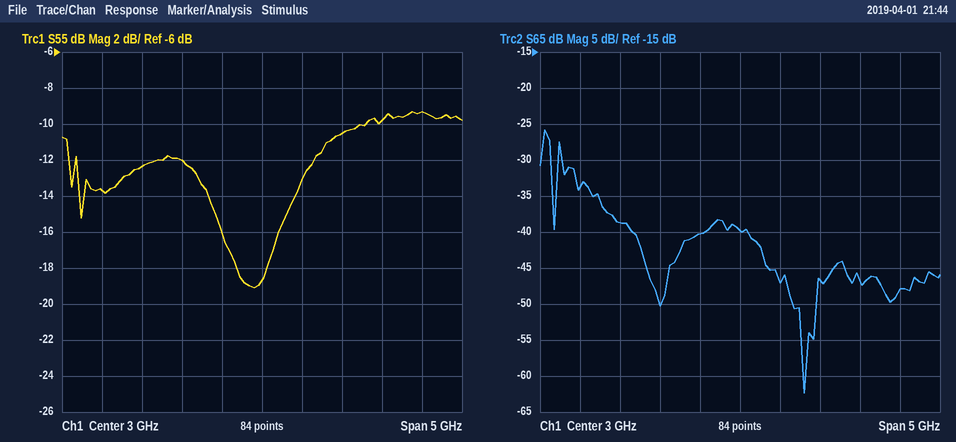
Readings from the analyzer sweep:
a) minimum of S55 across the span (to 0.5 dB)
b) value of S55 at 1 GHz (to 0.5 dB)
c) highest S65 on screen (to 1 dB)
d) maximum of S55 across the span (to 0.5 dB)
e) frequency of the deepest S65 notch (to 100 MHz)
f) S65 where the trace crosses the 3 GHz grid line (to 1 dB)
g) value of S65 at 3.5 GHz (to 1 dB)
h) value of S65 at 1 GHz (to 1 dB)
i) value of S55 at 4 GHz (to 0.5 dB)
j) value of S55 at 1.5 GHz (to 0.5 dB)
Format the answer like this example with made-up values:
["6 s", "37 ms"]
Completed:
["-19.0 dB", "-13.5 dB", "-26 dB", "-9.5 dB", "3.8 GHz", "-40 dB", "-47 dB", "-34 dB", "-10.5 dB", "-12.5 dB"]
